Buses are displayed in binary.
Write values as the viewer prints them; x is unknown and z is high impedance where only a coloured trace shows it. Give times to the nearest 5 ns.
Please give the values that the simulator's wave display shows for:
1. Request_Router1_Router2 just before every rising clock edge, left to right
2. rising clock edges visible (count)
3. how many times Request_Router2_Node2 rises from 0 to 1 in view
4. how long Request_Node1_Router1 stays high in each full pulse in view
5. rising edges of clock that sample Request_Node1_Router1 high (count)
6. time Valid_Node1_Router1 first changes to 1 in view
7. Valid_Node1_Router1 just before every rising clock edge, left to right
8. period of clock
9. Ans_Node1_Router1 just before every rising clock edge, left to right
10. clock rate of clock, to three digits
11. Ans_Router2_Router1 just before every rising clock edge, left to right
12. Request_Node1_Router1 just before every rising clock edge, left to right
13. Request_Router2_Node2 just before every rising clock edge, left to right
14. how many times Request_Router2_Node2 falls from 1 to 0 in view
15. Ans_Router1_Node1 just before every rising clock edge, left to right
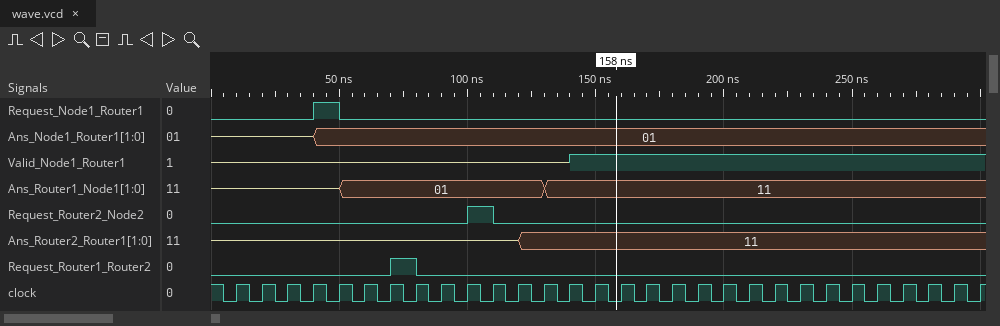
0 0 0 0 0 0 0 1 0 0 0 0 0 0 0 0 0 0 0 0 0 0 0 0 0 0 0 0 0 0
30
1
10 ns
1
140 ns
z z z z z z z z z z z z z z 1 1 1 1 1 1 1 1 1 1 1 1 1 1 1 1
10 ns
z, z, z, z, 01, 01, 01, 01, 01, 01, 01, 01, 01, 01, 01, 01, 01, 01, 01, 01, 01, 01, 01, 01, 01, 01, 01, 01, 01, 01
100 MHz
z, z, z, z, z, z, z, z, z, z, z, z, 11, 11, 11, 11, 11, 11, 11, 11, 11, 11, 11, 11, 11, 11, 11, 11, 11, 11
0 0 0 0 1 0 0 0 0 0 0 0 0 0 0 0 0 0 0 0 0 0 0 0 0 0 0 0 0 0
0 0 0 0 0 0 0 0 0 0 1 0 0 0 0 0 0 0 0 0 0 0 0 0 0 0 0 0 0 0
1
z, z, z, z, z, 01, 01, 01, 01, 01, 01, 01, 01, 11, 11, 11, 11, 11, 11, 11, 11, 11, 11, 11, 11, 11, 11, 11, 11, 11
